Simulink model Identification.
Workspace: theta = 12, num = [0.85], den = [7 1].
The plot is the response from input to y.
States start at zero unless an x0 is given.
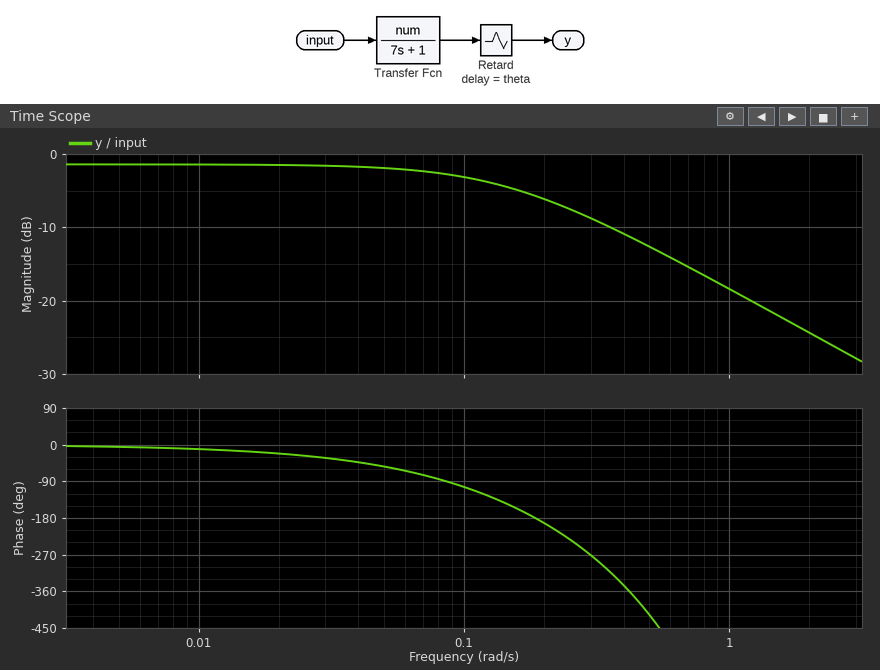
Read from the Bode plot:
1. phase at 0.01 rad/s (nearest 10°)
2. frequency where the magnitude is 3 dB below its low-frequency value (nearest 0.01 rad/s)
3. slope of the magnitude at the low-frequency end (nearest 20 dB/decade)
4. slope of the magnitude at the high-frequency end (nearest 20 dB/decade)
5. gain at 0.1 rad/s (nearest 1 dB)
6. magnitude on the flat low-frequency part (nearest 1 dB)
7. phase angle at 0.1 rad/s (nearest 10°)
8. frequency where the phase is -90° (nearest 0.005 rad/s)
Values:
-10°
0.14 rad/s
0 dB/decade
-20 dB/decade
-3 dB
-1 dB
-100°
0.085 rad/s
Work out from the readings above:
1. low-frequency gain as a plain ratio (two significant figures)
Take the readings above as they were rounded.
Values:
0.89
